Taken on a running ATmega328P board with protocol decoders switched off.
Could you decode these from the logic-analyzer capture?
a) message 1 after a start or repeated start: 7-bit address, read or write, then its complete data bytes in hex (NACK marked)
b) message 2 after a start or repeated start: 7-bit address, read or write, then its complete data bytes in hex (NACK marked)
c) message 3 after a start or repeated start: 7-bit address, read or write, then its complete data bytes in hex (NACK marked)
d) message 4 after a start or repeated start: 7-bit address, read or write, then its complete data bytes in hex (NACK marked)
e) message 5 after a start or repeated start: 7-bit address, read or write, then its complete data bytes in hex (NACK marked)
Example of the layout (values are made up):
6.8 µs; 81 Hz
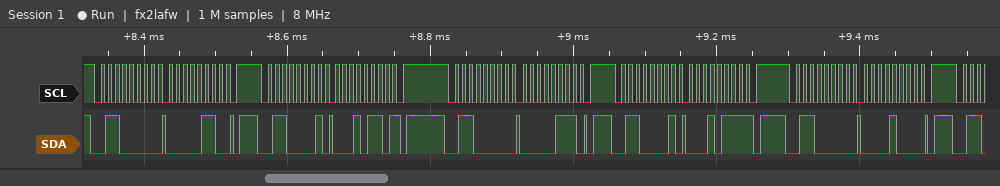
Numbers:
0x30 write: 06; 0x30 read: 16 NACK; 0x30 write: 07; 0x30 read: 17 NACK; 0x30 write: 08
